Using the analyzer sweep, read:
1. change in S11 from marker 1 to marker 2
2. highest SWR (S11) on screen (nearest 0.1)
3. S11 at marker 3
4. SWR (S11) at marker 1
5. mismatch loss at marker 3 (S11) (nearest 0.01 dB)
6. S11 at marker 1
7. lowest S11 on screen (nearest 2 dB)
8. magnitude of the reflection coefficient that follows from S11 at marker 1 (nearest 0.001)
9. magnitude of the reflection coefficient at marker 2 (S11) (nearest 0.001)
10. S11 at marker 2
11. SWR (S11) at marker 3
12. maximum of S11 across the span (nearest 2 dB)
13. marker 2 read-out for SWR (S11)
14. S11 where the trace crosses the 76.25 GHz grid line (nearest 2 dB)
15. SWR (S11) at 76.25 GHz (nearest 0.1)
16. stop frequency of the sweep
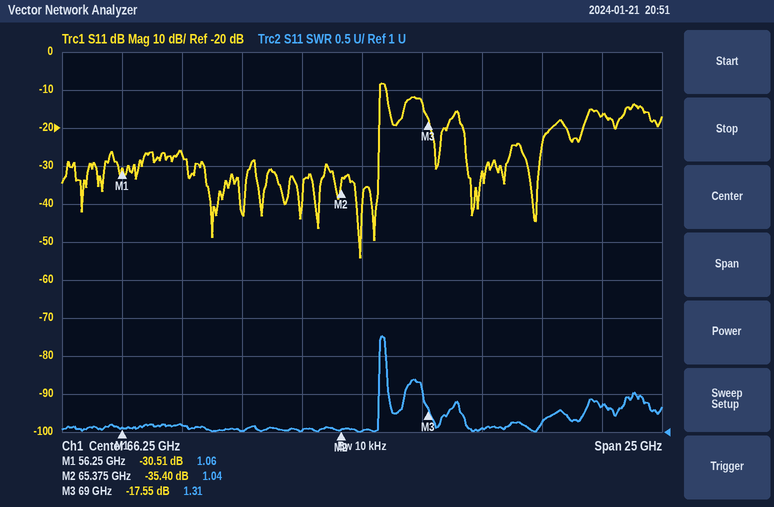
-4.89 dB
2.3
-17.55 dB
1.06
0.08 dB
-30.51 dB
-54 dB
0.030
0.017
-35.40 dB
1.31
-8 dB
1.04
-16 dB
1.3
78.75 GHz
